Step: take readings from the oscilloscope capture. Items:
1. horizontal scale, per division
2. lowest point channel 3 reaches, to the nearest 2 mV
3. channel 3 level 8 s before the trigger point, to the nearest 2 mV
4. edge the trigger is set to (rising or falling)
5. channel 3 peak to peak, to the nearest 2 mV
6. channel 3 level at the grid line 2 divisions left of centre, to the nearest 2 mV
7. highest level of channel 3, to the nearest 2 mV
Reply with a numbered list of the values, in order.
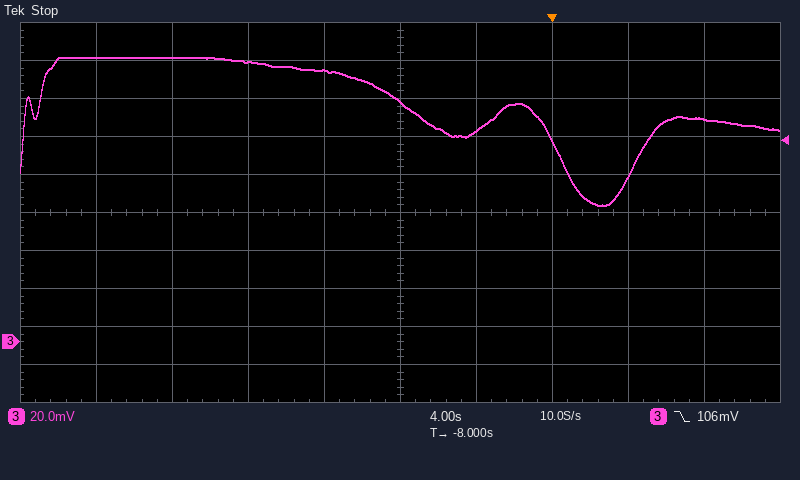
1. 4 s
2. 72 mV
3. 126 mV
4. falling
5. 78 mV
6. 148 mV
7. 150 mV
